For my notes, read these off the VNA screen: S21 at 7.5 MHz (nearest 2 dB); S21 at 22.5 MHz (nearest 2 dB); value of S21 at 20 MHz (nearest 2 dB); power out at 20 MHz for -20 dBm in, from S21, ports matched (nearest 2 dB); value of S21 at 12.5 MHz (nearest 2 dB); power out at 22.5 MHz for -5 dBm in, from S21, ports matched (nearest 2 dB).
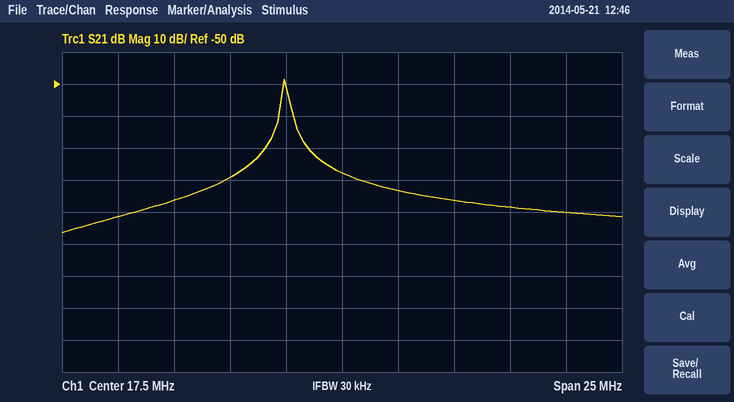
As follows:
-92 dB
-86 dB
-84 dB
-104 dBm
-80 dB
-92 dBm
